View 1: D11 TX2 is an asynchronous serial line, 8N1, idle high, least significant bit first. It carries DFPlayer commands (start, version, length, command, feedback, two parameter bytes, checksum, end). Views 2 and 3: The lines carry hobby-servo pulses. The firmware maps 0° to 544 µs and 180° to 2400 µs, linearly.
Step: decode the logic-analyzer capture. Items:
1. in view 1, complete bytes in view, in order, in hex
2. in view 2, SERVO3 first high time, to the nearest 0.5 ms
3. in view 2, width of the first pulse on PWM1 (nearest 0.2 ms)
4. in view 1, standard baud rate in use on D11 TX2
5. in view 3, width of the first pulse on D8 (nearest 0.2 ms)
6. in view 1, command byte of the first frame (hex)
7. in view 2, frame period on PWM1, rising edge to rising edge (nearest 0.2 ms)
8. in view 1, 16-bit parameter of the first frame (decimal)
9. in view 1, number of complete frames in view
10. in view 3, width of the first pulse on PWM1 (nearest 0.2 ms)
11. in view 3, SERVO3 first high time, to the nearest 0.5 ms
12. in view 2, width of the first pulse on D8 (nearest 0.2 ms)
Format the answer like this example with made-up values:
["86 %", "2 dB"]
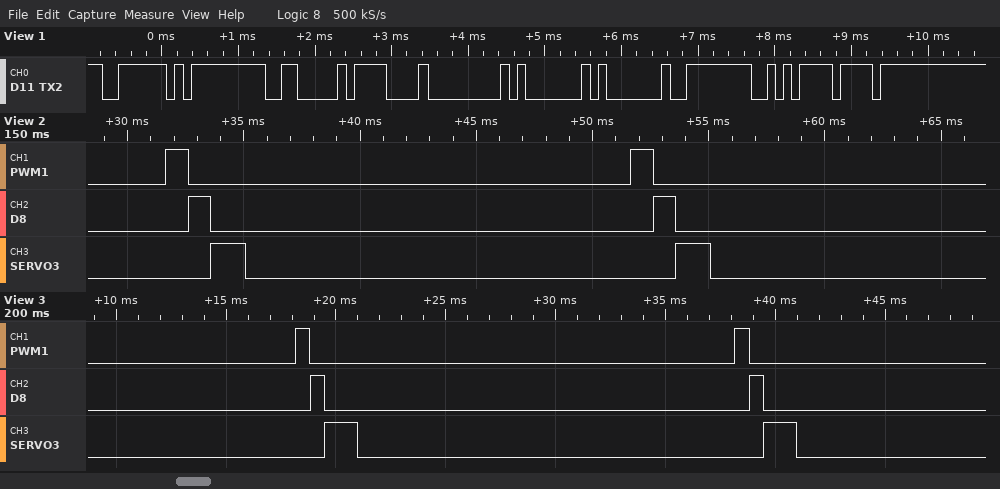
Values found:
["7E FF 06 0F 00 01 01 FE EA EF", "1.5 ms", "1.0 ms", "9600 baud", "0.6 ms", "0x0F", "20.0 ms", "257", "10", "0.6 ms", "1.5 ms", "1.0 ms"]
